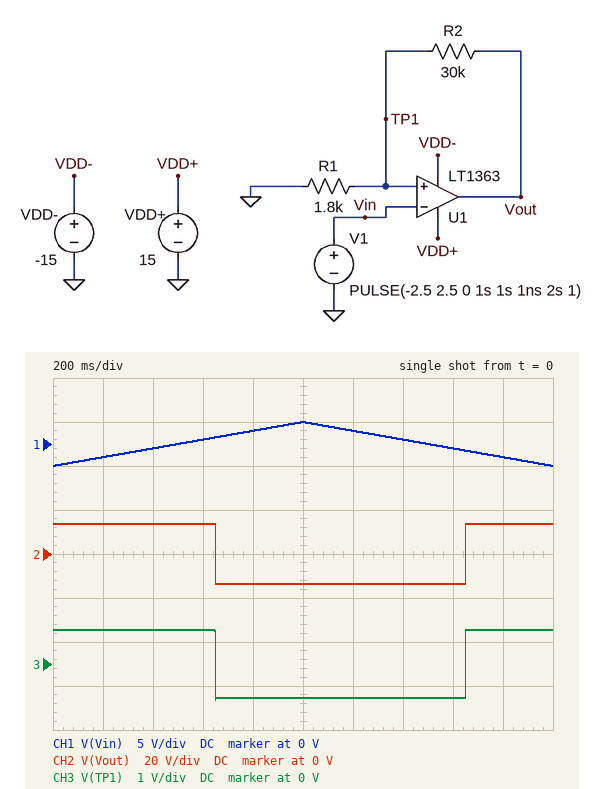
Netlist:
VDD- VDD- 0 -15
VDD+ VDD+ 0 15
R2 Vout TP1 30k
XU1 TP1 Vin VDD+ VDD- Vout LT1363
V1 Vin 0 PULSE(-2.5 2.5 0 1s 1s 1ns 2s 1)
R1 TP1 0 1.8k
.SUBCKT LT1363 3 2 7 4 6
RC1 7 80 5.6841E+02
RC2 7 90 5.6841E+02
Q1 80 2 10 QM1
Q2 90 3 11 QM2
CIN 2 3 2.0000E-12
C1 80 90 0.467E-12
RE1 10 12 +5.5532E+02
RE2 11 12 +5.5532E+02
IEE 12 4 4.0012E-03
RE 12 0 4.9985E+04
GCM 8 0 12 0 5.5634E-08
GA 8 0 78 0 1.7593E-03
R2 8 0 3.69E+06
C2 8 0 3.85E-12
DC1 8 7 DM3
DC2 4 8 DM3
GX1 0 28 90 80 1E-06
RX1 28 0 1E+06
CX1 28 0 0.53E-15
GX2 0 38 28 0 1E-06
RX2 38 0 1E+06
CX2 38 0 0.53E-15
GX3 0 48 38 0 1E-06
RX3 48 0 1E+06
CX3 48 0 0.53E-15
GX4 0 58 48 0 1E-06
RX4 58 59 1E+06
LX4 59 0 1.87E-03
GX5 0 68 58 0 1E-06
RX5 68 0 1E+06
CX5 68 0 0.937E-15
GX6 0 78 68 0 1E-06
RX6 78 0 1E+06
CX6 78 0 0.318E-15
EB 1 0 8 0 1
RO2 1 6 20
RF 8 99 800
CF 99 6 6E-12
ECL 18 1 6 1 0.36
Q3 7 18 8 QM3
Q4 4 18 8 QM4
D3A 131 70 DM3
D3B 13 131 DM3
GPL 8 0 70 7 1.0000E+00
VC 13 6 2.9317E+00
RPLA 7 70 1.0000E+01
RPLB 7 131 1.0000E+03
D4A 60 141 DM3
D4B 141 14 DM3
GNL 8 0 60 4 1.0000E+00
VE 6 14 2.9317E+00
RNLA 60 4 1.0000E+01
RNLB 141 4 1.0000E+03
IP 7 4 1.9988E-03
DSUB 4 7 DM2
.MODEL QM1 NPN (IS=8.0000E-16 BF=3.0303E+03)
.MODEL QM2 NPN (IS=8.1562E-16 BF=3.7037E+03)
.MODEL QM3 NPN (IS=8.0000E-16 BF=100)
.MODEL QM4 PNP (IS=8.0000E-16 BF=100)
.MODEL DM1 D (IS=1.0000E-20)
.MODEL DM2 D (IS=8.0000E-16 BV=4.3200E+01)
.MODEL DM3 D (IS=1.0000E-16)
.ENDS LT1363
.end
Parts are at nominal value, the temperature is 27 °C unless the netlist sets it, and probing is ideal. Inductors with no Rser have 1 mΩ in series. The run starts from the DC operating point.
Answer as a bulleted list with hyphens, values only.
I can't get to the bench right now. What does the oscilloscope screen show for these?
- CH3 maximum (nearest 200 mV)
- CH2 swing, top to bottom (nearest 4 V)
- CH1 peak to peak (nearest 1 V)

- 800 mV
- 28 V
- 5 V
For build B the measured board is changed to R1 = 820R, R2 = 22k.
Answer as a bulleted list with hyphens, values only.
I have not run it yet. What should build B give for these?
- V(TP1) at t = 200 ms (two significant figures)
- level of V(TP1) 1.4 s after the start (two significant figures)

- 490 mV
- -490 mV
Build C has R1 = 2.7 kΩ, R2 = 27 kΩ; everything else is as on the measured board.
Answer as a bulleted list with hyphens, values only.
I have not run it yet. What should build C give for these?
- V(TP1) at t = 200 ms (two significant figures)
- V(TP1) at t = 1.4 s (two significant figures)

- 1.2 V
- -1.2 V
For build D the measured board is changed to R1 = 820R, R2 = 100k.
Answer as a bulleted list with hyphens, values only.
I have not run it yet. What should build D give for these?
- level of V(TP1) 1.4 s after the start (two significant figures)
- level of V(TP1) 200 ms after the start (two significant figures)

- -110 mV
- 110 mV
